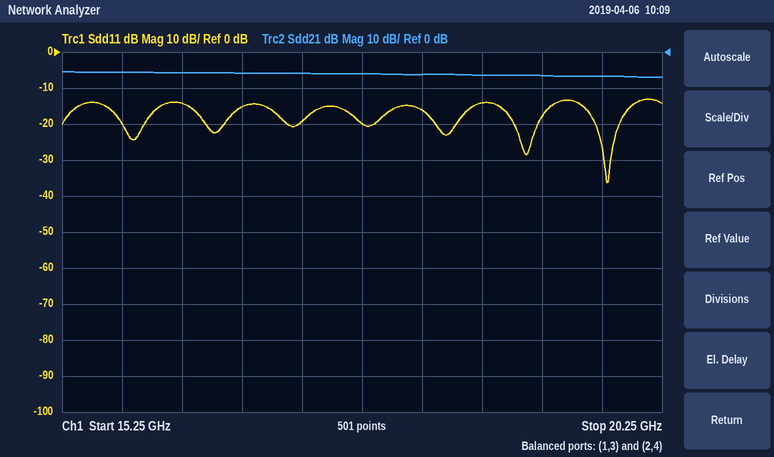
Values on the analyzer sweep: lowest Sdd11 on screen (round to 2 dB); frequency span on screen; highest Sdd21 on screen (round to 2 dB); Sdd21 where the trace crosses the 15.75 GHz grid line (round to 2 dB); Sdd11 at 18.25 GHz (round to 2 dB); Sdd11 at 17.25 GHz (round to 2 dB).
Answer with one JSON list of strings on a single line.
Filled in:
["-36 dB", "5 GHz", "-6 dB", "-6 dB", "-16 dB", "-20 dB"]
